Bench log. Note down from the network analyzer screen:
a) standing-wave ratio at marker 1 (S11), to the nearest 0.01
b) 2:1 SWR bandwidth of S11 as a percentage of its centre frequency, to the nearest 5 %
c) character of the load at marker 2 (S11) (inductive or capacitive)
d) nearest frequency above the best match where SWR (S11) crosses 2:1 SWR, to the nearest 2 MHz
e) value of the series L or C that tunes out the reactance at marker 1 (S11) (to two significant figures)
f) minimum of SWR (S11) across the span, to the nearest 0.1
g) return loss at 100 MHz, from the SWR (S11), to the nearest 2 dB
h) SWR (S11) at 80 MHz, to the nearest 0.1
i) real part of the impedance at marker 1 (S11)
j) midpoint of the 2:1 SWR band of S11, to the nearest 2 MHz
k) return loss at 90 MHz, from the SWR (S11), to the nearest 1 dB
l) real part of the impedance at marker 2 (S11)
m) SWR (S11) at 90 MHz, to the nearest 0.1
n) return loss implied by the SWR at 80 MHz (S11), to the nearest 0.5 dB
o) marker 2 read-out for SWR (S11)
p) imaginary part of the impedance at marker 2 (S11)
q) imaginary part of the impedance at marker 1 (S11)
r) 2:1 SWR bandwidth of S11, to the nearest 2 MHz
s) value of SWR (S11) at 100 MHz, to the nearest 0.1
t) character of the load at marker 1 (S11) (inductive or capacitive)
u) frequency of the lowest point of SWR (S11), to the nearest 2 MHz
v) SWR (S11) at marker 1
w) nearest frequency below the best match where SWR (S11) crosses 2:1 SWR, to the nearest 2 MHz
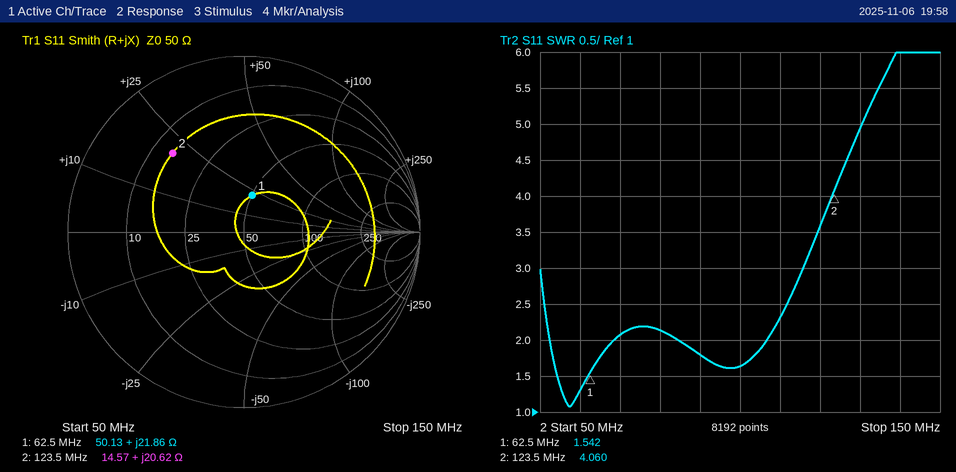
1.54
25 %
inductive
68 MHz
120 pF
1.1
12 dB
2.1
50.13 Ω
60 MHz
11 dB
14.57 Ω
1.8
9.0 dB
4.060
+20.62 Ω
+21.86 Ω
16 MHz
1.6
inductive
58 MHz
1.542
52 MHz
